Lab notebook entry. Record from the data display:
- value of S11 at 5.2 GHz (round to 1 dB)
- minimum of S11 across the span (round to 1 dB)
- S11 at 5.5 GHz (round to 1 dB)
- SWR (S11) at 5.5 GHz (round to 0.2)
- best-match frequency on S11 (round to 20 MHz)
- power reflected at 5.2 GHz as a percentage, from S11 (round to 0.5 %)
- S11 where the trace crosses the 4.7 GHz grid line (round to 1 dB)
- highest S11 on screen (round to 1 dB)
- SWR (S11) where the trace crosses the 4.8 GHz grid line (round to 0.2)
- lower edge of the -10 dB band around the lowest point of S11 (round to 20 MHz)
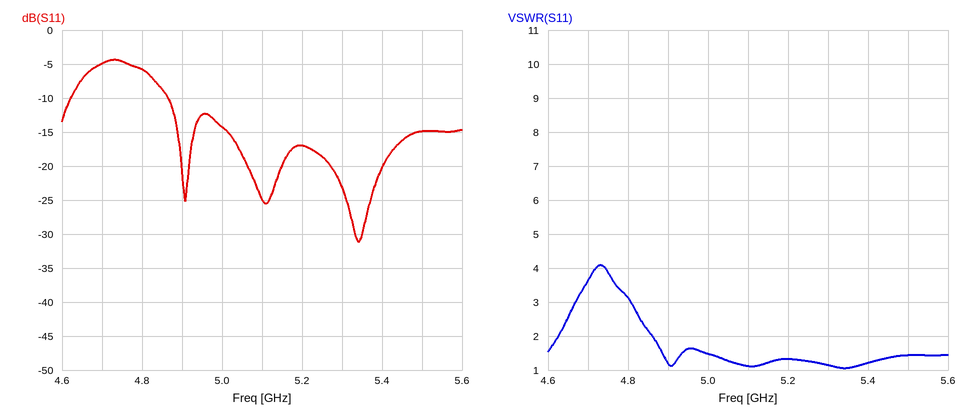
-17 dB
-31 dB
-15 dB
1.4
5.34 GHz
2.0 %
-5 dB
-4 dB
3.2
4.86 GHz
